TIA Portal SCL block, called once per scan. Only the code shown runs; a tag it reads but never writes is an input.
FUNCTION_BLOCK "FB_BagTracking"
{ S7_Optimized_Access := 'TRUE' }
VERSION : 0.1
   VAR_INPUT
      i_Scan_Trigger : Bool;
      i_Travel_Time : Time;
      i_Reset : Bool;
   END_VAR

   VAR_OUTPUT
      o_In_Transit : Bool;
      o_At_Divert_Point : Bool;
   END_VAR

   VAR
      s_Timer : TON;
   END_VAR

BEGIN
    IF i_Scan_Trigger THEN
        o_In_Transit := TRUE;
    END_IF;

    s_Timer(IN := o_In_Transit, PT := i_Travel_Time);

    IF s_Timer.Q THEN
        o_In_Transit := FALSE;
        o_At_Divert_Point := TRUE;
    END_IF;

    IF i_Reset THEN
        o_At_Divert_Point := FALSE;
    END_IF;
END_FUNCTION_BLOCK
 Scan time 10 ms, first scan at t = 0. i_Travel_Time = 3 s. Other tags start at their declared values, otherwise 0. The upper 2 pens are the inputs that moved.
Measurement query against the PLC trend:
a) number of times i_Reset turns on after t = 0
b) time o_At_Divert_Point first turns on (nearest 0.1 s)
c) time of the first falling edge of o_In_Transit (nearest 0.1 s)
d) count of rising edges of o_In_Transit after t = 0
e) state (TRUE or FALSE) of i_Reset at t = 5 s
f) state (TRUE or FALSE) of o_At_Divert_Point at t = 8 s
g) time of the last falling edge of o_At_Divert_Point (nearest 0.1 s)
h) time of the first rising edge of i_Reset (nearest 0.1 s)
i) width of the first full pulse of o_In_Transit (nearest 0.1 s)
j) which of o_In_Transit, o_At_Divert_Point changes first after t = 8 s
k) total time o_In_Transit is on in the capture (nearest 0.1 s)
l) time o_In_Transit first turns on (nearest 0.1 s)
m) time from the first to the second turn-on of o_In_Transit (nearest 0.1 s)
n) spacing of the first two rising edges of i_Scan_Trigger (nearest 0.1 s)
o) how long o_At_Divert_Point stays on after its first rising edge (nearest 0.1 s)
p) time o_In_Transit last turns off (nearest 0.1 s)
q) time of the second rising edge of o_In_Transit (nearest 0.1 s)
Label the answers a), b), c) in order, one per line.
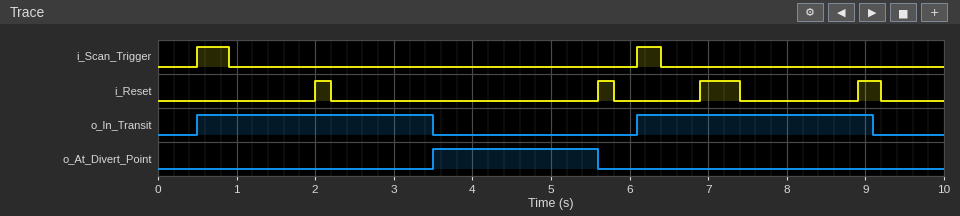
a) 4
b) 3.5 s
c) 3.5 s
d) 2
e) FALSE
f) FALSE
g) 5.6 s
h) 2.0 s
i) 3.0 s
j) o_In_Transit
k) 6.0 s
l) 0.5 s
m) 5.6 s
n) 5.6 s
o) 2.1 s
p) 9.1 s
q) 6.1 s
